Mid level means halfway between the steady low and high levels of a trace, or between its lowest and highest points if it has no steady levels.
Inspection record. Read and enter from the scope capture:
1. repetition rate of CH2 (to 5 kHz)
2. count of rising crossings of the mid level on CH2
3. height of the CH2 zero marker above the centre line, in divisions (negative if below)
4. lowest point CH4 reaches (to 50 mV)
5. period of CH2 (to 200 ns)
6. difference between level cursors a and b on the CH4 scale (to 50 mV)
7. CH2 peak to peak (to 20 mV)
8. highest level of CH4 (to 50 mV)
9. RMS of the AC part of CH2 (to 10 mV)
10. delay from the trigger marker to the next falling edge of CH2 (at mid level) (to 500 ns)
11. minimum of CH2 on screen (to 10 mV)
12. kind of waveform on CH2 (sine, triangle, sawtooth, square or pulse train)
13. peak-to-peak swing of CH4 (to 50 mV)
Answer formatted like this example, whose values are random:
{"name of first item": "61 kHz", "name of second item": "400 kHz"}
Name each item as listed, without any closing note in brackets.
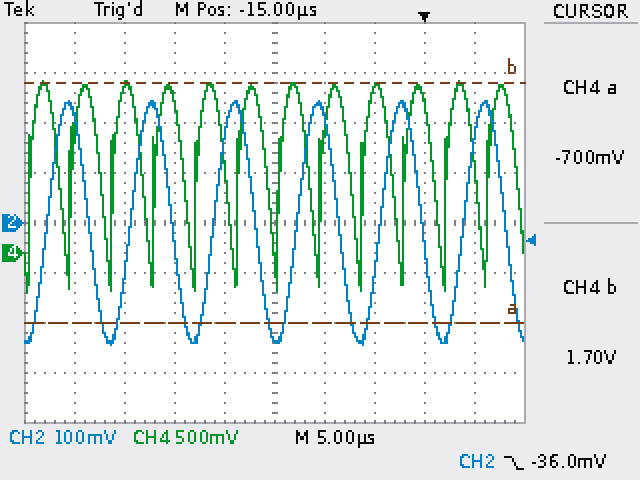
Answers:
{"repetition rate of CH2": "120 kHz", "count of rising crossings of the mid level on CH2": "6", "height of the CH2 zero marker above the centre line, in divisions": "0.0 div", "lowest point CH4 reaches": "-400 mV", "period of CH2": "8.4 µs", "difference between level cursors a and b on the CH4 scale": "2.40 V", "CH2 peak to peak": "480 mV", "highest level of CH4": "1.70 V", "RMS of the AC part of CH2": "170 mV", "delay from the trigger marker to the next falling edge of CH2 (at mid level)": "8.0 µs", "minimum of CH2 on screen": "-240 mV", "kind of waveform on CH2": "sine", "peak-to-peak swing of CH4": "2.10 V"}
